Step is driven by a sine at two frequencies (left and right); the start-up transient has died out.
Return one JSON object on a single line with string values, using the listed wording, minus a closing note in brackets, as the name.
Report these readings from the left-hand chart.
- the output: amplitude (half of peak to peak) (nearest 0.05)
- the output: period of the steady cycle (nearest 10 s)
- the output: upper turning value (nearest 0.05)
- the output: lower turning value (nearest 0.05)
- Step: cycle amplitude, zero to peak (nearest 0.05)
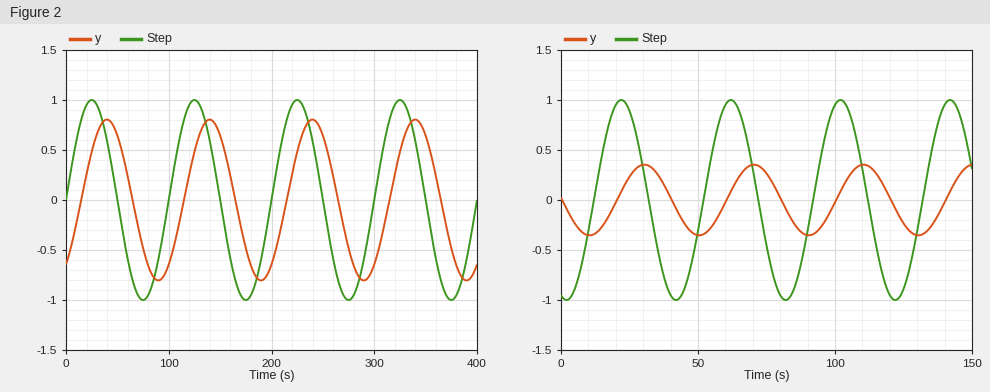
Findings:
{"the output: amplitude (half of peak to peak)": "0.80", "the output: period of the steady cycle": "100 s", "the output: upper turning value": "0.80", "the output: lower turning value": "-0.80", "Step: cycle amplitude, zero to peak": "1.00"}
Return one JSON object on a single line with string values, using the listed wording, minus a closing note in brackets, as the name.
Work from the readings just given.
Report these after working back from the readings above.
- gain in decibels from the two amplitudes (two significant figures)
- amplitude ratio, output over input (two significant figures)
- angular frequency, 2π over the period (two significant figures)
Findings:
{"gain in decibels from the two amplitudes": "-1.9 dB", "amplitude ratio, output over input": "0.80", "angular frequency, 2π over the period": "0.063 rad/s"}
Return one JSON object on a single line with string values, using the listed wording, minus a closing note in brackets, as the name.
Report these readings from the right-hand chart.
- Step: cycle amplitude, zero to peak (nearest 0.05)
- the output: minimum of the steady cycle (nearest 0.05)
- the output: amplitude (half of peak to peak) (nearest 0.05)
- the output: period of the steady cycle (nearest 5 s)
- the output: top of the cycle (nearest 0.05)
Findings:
{"Step: cycle amplitude, zero to peak": "1.00", "the output: minimum of the steady cycle": "-0.35", "the output: amplitude (half of peak to peak)": "0.35", "the output: period of the steady cycle": "40 s", "the output: top of the cycle": "0.35"}
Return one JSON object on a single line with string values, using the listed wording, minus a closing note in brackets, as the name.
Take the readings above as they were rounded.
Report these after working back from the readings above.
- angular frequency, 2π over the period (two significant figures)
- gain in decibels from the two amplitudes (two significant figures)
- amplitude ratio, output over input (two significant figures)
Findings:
{"angular frequency, 2π over the period": "0.16 rad/s", "gain in decibels from the two amplitudes": "-9.1 dB", "amplitude ratio, output over input": "0.35"}
